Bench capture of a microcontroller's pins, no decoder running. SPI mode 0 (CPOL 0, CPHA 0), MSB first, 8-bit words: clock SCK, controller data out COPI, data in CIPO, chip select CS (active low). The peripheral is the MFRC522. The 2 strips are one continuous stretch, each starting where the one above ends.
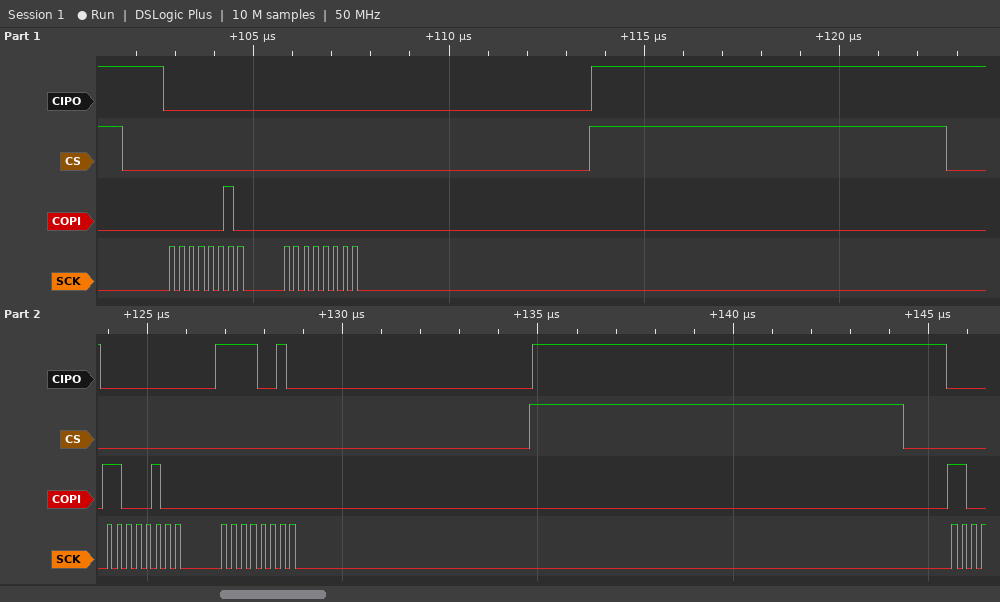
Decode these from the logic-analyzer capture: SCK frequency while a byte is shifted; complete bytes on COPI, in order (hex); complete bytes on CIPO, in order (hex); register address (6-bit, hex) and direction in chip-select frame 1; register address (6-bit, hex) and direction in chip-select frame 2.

4 MHz
02 00 C4 00
00 00 00 F2
0x01 write
0x22 read
